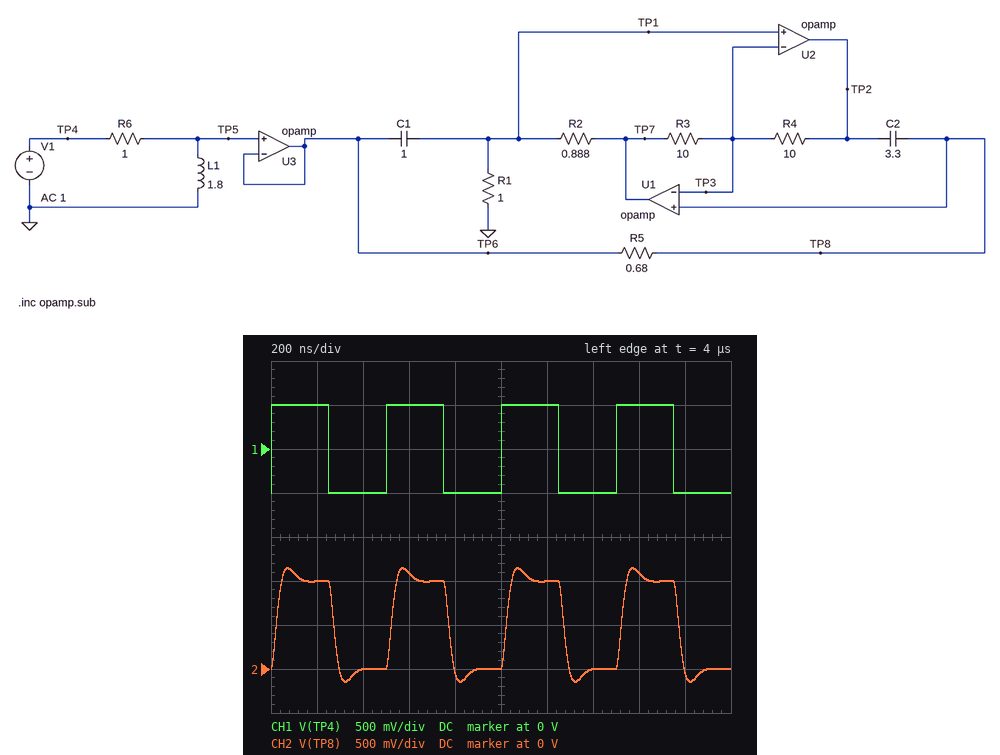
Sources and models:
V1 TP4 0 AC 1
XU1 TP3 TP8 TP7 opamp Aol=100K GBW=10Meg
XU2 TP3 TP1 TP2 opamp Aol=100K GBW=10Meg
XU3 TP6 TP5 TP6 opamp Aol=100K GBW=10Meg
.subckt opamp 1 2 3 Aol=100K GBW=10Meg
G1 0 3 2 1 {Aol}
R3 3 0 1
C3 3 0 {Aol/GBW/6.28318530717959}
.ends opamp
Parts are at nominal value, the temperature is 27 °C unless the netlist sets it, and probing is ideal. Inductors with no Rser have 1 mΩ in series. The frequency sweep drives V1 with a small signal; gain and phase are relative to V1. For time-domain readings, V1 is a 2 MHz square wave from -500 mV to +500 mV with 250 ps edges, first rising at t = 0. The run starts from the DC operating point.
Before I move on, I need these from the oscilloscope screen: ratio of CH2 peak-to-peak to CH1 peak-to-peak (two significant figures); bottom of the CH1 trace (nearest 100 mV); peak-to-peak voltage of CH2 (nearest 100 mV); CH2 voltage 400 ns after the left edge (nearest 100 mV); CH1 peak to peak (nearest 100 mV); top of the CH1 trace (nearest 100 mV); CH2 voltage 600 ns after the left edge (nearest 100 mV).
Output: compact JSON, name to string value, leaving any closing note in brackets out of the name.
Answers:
{"ratio of CH2 peak-to-peak to CH1 peak-to-peak": "1.3", "bottom of the CH1 trace": "-500 mV", "peak-to-peak voltage of CH2": "1.3 V", "CH2 voltage 400 ns after the left edge": "0 V", "CH1 peak to peak": "1.0 V", "top of the CH1 trace": "500 mV", "CH2 voltage 600 ns after the left edge": "1.1 V"}
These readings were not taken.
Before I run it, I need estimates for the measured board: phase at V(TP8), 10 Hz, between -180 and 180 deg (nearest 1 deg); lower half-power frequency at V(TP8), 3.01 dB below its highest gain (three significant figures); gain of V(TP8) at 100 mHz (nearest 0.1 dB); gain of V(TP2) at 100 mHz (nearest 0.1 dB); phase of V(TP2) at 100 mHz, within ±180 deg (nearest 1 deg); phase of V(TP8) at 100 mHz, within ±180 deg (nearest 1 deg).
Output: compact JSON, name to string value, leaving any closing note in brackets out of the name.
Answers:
{"phase at V(TP8), 10 Hz, between -180 and 180 deg": "1 deg", "lower half-power frequency at V(TP8), 3.01 dB below its highest gain": "237 mHz", "gain of V(TP8) at 100 mHz": "-18.0 dB", "gain of V(TP2) at 100 mHz": "-8.0 dB", "phase of V(TP2) at 100 mHz, within ±180 deg": "141 deg", "phase of V(TP8) at 100 mHz, within ±180 deg": "-39 deg"}
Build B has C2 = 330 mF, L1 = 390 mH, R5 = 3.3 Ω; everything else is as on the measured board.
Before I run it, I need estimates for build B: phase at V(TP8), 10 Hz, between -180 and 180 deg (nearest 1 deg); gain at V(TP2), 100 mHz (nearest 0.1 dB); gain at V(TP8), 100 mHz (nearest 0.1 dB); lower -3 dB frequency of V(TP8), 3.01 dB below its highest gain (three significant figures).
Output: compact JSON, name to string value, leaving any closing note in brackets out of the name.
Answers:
{"phase at V(TP8), 10 Hz, between -180 and 180 deg": "3 deg", "gain at V(TP2), 100 mHz": "-22.6 dB", "gain at V(TP8), 100 mHz": "-15.4 dB", "lower -3 dB frequency of V(TP8), 3.01 dB below its highest gain": "473 mHz"}
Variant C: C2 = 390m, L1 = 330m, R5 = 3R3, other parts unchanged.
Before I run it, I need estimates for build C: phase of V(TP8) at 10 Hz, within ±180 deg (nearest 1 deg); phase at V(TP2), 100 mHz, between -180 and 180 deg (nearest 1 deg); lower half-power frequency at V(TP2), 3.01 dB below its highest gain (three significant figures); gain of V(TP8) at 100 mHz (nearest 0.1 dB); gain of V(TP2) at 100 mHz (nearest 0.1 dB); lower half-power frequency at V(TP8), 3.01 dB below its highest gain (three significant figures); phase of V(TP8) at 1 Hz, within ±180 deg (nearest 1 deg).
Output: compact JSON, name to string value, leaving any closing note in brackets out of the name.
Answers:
{"phase of V(TP8) at 10 Hz, within ±180 deg": "4 deg", "phase at V(TP2), 100 mHz, between -180 and 180 deg": "-155 deg", "lower half-power frequency at V(TP2), 3.01 dB below its highest gain": "456 mHz", "gain of V(TP8) at 100 mHz": "-18.2 dB", "gain of V(TP2) at 100 mHz": "-22.4 dB", "lower half-power frequency at V(TP8), 3.01 dB below its highest gain": "536 mHz", "phase of V(TP8) at 1 Hz, within ±180 deg": "35 deg"}
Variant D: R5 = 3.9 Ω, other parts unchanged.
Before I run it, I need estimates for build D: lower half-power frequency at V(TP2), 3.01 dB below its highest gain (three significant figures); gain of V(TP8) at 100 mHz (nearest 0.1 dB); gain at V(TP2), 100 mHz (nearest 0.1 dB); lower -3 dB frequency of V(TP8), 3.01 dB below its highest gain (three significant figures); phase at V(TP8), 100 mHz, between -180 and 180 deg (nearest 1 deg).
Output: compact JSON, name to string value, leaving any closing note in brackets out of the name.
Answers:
{"lower half-power frequency at V(TP2), 3.01 dB below its highest gain": "186 mHz", "gain of V(TP8) at 100 mHz": "-9.7 dB", "gain at V(TP2), 100 mHz": "-7.7 dB", "lower -3 dB frequency of V(TP8), 3.01 dB below its highest gain": "204 mHz", "phase at V(TP8), 100 mHz, between -180 and 180 deg": "105 deg"}
